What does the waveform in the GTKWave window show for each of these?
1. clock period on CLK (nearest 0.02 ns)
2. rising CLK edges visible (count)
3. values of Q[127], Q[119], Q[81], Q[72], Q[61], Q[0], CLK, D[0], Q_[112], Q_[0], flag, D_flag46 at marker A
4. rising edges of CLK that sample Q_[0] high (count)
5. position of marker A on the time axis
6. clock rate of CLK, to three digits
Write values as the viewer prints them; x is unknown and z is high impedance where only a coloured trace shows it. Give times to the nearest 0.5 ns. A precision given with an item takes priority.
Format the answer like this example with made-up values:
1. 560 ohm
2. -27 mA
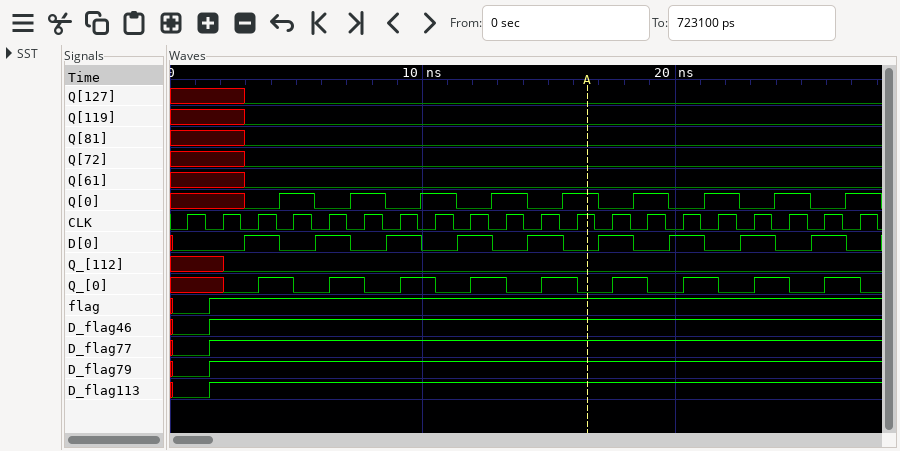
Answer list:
1. 1.4 ns
2. 20
3. Q[127]=0, Q[119]=0, Q[81]=0, Q[72]=0, Q[61]=0, Q[0]=1, CLK=1, D[0]=0, Q_[112]=0, Q_[0]=0, flag=1, D_flag46=1
4. 9
5. 16.5 ns
6. 714 MHz
